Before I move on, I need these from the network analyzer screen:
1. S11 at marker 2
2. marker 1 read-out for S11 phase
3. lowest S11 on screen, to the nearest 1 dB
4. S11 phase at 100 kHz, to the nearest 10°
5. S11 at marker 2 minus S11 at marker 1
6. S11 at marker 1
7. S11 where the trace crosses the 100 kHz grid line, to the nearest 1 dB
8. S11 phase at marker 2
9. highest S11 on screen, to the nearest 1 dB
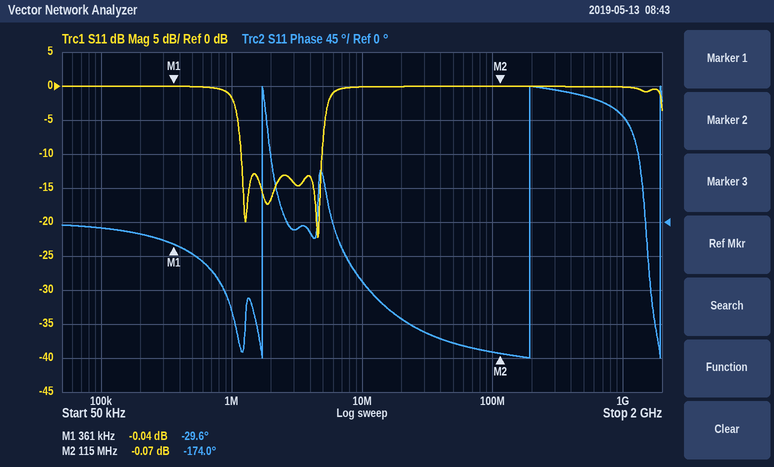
-0.07 dB
-29.6°
-22 dB
-10°
-0.03 dB
-0.04 dB
0 dB
-174.0°
0 dB
